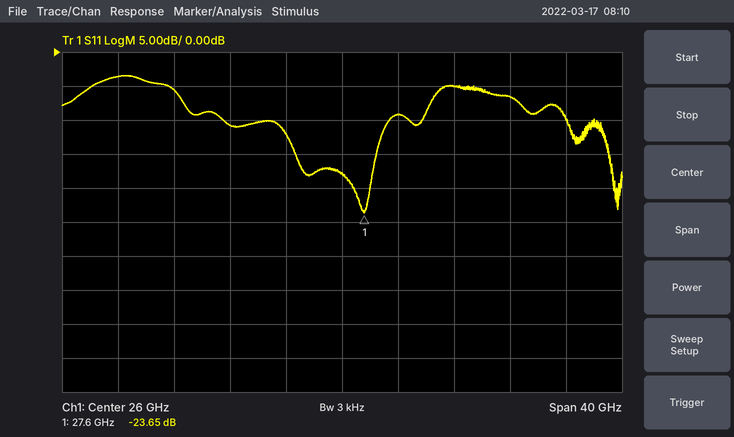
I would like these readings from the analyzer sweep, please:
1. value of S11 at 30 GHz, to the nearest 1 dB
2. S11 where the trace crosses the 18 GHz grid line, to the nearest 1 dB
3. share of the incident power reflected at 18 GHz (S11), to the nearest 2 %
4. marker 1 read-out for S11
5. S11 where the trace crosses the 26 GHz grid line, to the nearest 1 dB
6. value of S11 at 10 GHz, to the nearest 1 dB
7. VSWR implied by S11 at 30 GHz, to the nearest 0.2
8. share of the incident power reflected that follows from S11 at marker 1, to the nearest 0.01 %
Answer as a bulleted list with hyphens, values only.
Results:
- -9 dB
- -11 dB
- 8 %
- -23.65 dB
- -18 dB
- -4 dB
- 2.0
- 0.43 %
